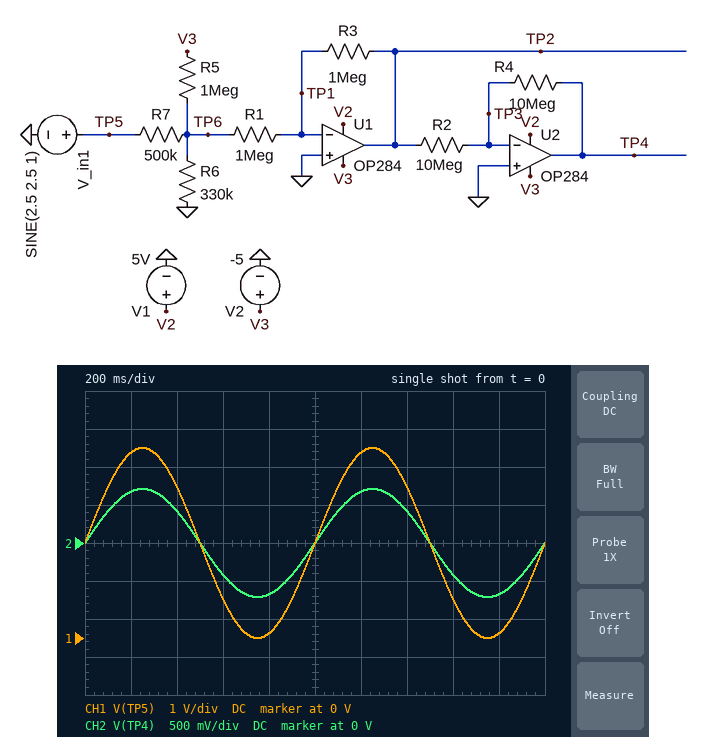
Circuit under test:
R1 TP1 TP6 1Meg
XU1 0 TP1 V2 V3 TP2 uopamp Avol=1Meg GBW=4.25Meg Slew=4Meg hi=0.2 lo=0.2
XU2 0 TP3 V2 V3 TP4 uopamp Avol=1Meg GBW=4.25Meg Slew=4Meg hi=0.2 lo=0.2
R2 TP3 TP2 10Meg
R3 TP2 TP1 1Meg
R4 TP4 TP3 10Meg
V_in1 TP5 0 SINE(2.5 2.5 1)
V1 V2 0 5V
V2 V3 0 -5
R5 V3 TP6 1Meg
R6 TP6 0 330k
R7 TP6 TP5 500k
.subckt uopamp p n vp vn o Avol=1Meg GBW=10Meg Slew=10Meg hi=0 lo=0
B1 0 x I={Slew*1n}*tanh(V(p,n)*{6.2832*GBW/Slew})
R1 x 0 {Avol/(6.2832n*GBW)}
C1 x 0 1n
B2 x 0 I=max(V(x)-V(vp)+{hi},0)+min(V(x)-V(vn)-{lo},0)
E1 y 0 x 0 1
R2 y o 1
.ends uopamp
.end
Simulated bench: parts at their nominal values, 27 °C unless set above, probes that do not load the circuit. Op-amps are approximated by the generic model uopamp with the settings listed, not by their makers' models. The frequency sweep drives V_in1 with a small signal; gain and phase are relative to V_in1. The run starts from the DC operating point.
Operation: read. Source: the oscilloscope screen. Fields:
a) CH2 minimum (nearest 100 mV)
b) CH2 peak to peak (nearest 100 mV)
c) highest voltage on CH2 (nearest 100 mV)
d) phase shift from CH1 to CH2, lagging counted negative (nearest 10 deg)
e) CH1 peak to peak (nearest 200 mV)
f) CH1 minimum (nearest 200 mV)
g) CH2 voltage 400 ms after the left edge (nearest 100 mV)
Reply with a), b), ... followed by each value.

a) -700 mV
b) 1.4 V
c) 700 mV
d) 0 deg
e) 5.0 V
f) 0 V
g) 400 mV
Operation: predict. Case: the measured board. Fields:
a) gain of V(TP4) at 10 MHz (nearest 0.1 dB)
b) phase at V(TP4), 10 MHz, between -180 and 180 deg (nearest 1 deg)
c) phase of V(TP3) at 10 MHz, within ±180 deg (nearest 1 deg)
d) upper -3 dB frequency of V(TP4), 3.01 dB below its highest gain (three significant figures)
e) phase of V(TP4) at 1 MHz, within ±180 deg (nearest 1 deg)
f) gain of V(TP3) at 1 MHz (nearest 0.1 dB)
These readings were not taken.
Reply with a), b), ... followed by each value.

a) -37.6 dB
b) -155 deg
c) 115 deg
d) 1.42 MHz
e) -49 deg
f) -25.1 dB
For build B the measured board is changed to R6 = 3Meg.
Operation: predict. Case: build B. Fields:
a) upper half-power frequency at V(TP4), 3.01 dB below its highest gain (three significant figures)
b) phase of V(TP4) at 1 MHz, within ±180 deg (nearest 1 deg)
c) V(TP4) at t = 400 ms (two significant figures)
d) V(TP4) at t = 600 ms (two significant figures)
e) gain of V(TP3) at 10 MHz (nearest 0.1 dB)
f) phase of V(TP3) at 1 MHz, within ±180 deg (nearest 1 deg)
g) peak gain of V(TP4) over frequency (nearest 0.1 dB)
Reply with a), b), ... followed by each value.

a) 1.45 MHz
b) -48 deg
c) 680 mV
d) -680 mV
e) -25.6 dB
f) -138 deg
g) -6.7 dB
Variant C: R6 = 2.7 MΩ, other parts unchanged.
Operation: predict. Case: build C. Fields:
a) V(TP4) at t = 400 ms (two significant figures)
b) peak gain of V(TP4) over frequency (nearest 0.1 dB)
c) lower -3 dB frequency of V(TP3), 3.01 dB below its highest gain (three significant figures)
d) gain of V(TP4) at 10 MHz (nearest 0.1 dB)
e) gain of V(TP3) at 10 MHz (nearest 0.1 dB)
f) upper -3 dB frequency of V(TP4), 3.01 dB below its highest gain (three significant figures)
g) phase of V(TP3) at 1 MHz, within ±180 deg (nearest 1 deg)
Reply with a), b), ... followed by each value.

a) 670 mV
b) -6.8 dB
c) 934 kHz
d) -33.1 dB
e) -25.6 dB
f) 1.45 MHz
g) -138 deg
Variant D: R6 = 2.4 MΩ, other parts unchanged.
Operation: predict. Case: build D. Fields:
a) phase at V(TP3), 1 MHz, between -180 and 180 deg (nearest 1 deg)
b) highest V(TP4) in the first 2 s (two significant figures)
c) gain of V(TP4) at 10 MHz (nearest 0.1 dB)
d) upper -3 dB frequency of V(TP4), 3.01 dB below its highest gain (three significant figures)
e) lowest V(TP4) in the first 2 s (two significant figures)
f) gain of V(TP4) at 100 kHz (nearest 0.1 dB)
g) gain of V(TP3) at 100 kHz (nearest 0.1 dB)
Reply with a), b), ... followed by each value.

a) -138 deg
b) 1.1 V
c) -33.2 dB
d) 1.45 MHz
e) -1.1 V
f) -6.9 dB
g) -39.5 dB
